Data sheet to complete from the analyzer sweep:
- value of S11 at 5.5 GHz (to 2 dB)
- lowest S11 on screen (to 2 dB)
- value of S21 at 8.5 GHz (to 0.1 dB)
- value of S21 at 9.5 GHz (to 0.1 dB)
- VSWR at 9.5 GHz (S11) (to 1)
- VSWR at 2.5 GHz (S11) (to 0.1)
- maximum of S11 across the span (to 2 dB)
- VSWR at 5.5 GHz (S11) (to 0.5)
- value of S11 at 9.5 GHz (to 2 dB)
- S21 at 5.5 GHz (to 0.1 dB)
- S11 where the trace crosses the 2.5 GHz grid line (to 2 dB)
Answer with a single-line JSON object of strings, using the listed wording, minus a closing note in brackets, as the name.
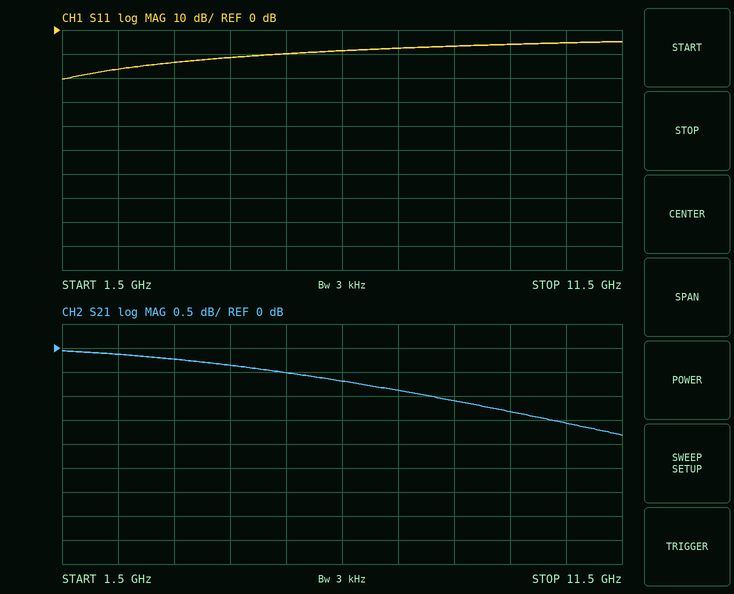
{"value of S11 at 5.5 GHz": "-10 dB", "lowest S11 on screen": "-20 dB", "value of S21 at 8.5 GHz": "-1.1 dB", "value of S21 at 9.5 GHz": "-1.3 dB", "VSWR at 9.5 GHz (S11)": "3", "VSWR at 2.5 GHz (S11)": "1.4", "maximum of S11 across the span": "-4 dB", "VSWR at 5.5 GHz (S11)": "2.0", "value of S11 at 9.5 GHz": "-6 dB", "S21 at 5.5 GHz": "-0.5 dB", "S11 where the trace crosses the 2.5 GHz grid line": "-16 dB"}
